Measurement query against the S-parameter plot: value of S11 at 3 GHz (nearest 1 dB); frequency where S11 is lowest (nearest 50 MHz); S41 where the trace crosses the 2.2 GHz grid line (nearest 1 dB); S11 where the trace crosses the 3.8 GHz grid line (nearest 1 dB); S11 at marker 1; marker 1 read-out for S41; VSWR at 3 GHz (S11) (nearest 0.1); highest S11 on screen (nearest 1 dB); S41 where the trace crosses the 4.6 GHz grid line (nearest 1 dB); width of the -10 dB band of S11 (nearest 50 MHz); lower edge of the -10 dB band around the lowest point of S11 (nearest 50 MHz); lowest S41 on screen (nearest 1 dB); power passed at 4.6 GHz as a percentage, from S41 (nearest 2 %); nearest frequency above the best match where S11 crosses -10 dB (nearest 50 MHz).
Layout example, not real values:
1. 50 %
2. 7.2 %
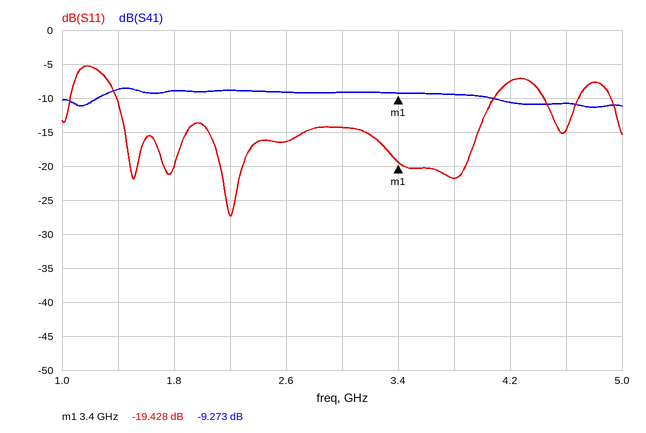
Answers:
1. -14 dB
2. 2.20 GHz
3. -9 dB
4. -22 dB
5. -19.428 dB
6. -9.273 dB
7. 1.5
8. -5 dB
9. -11 dB
10. 2.70 GHz
11. 1.40 GHz
12. -11 dB
13. 8 %
14. 4.10 GHz
